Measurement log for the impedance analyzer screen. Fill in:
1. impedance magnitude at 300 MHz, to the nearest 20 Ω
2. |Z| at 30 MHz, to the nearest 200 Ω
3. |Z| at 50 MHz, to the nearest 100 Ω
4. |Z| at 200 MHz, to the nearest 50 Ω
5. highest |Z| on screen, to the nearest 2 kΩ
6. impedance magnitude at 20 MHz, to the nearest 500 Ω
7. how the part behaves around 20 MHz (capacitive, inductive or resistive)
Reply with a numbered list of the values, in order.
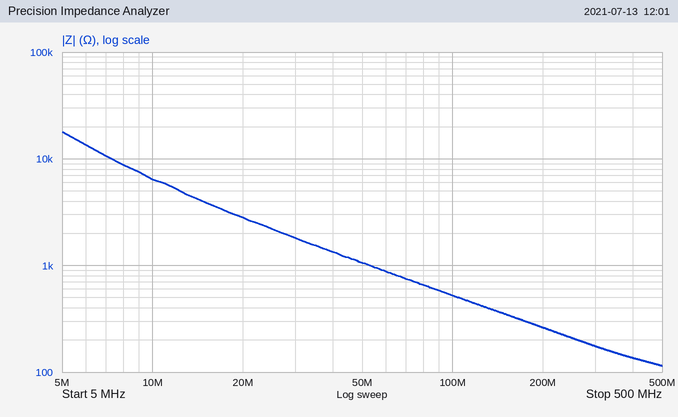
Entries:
1. 180 Ω
2. 1.8 kΩ
3. 1.1 kΩ
4. 250 Ω
5. 18 kΩ
6. 3.0 kΩ
7. capacitive
